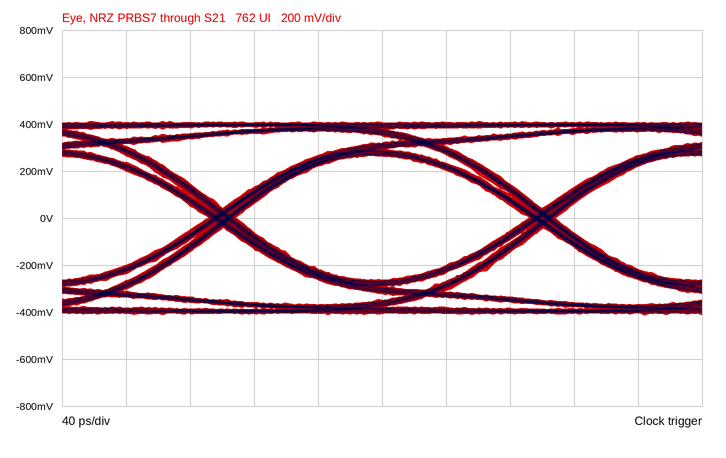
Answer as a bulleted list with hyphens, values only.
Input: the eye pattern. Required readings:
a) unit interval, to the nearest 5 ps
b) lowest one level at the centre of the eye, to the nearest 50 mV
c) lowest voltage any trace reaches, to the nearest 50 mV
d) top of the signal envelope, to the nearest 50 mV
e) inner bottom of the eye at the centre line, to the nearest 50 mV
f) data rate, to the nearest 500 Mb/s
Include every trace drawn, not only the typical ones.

- 200 ps
- 250 mV
- -400 mV
- 400 mV
- -250 mV
- 5.0 Gb/s
